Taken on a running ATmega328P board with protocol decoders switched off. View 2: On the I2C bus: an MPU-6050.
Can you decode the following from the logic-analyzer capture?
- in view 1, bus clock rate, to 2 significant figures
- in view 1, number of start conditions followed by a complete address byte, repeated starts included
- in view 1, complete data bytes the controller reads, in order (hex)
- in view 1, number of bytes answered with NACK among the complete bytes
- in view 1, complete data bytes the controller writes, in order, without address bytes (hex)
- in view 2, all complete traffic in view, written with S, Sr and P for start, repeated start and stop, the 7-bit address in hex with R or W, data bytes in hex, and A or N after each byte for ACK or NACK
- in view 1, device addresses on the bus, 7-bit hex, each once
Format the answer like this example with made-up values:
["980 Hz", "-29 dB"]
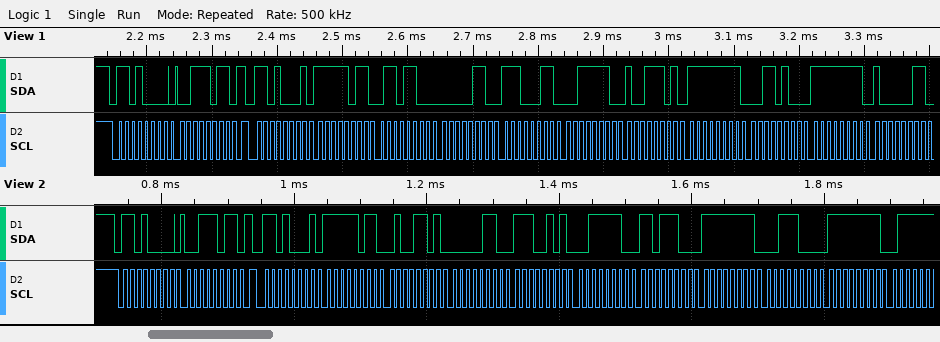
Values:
["100 kHz", "2", "FB 6C 06 E3 3E 9D FF 34 FF 83", "0", "3B", "S 68W A 3B A Sr 68R A FB A 4D A 06 A E5 A 3E A DC A FF A 38 A FF A", "0x68"]
